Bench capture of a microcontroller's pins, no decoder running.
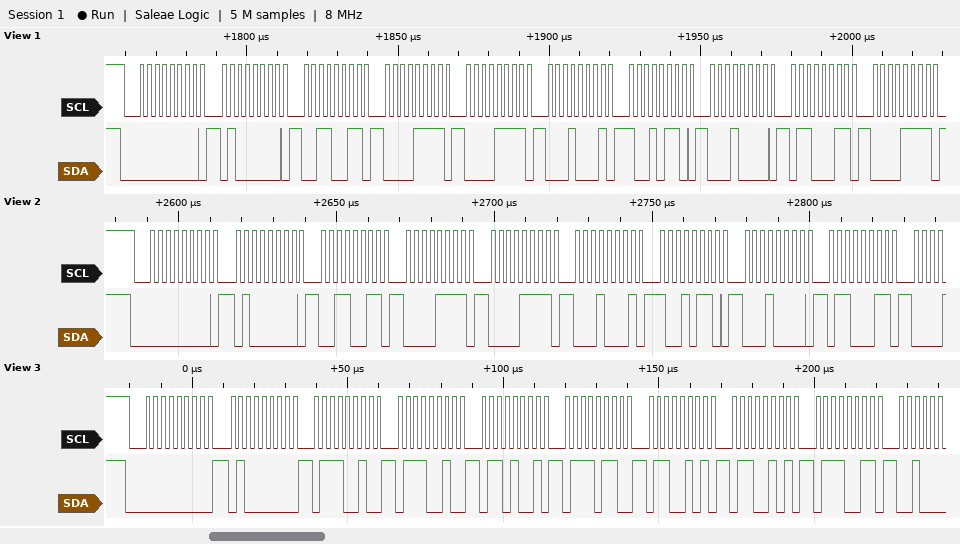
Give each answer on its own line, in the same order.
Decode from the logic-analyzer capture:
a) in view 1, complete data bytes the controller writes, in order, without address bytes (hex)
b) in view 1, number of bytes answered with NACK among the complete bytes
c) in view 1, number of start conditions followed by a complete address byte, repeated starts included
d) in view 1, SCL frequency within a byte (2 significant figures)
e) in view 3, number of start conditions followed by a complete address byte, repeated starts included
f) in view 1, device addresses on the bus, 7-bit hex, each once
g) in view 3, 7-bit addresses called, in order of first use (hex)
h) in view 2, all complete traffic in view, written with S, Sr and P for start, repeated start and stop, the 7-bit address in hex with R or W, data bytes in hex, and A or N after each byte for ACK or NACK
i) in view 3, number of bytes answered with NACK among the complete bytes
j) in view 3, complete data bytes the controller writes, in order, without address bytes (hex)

40 33 0F 0F 11 96 10 63 0F
0
1
400 kHz
1
0x00
0x00
S 00W A 40 A 33 A 0F A 0F A 11 A 96 A 10 A 63 A
0
40 72 72 69 76 65 65 73
